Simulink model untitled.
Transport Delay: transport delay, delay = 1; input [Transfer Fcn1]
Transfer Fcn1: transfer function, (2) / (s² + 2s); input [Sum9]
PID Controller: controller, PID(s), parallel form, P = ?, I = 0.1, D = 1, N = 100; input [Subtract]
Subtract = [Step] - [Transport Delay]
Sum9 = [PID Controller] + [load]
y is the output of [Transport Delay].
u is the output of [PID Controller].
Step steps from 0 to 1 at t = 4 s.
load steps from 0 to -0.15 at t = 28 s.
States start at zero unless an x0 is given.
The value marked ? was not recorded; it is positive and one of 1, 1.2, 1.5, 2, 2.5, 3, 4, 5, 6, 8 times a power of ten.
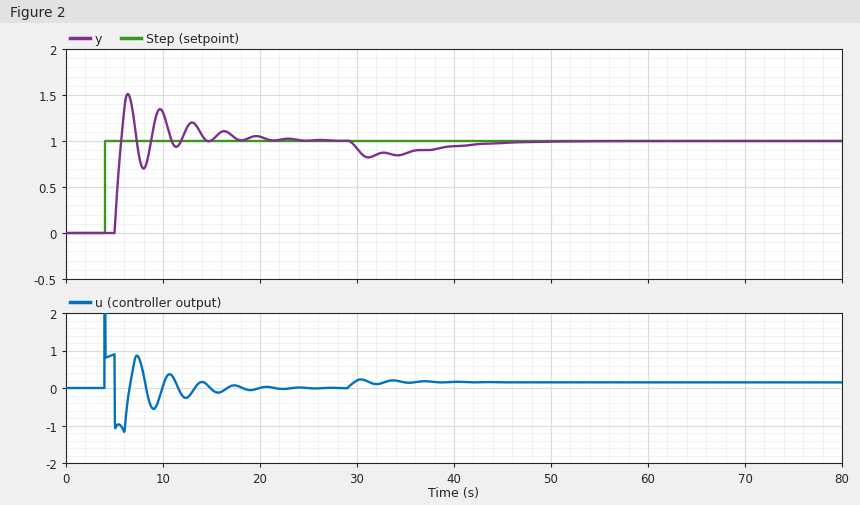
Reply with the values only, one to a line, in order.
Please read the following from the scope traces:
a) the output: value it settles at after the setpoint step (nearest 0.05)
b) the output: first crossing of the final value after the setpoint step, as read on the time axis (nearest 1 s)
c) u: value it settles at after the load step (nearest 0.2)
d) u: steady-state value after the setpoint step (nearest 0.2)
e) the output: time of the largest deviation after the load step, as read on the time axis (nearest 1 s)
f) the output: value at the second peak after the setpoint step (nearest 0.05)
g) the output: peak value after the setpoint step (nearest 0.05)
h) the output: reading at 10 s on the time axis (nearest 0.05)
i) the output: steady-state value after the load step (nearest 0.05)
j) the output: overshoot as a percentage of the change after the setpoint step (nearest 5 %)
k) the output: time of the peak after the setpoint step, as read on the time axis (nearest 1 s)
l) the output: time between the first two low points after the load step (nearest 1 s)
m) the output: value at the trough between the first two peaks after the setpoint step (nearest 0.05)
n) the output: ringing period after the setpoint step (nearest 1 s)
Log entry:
1.00
6 s
0.2
0.0
31 s
1.35
1.50
1.30
1.00
50 %
6 s
3 s
0.70
3 s
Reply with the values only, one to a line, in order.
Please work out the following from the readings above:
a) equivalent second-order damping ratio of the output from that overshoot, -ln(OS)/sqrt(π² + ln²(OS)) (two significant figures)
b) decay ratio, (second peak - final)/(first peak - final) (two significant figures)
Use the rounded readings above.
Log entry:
0.22
0.70
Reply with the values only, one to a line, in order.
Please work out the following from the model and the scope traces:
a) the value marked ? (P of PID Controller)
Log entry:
0.8
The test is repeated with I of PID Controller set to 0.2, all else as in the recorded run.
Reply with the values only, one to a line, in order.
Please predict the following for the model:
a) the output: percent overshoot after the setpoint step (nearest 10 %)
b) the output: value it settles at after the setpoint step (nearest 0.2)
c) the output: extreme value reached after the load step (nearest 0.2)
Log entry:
60 %
1.0
0.8
